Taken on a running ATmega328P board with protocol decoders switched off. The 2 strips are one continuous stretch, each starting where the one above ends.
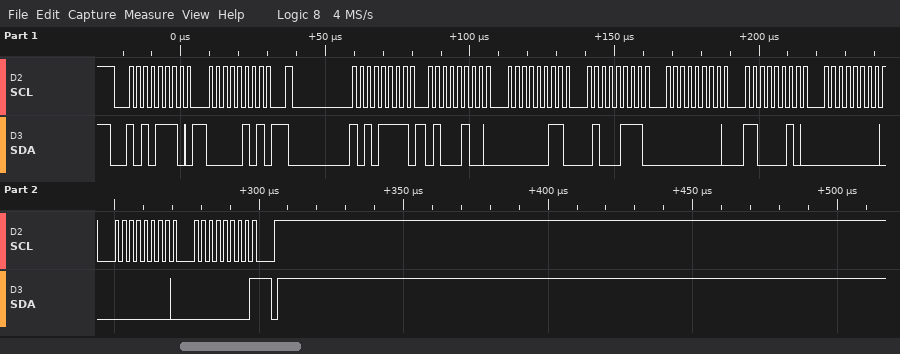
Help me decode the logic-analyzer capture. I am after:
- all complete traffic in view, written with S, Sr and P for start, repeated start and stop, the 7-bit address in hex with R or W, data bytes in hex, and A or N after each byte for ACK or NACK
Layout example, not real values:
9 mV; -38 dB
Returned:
S 57W A 05 A Sr 57R A 44 A 03 A 47 A 00 A C2 A 00 A 00 A 00 N P
